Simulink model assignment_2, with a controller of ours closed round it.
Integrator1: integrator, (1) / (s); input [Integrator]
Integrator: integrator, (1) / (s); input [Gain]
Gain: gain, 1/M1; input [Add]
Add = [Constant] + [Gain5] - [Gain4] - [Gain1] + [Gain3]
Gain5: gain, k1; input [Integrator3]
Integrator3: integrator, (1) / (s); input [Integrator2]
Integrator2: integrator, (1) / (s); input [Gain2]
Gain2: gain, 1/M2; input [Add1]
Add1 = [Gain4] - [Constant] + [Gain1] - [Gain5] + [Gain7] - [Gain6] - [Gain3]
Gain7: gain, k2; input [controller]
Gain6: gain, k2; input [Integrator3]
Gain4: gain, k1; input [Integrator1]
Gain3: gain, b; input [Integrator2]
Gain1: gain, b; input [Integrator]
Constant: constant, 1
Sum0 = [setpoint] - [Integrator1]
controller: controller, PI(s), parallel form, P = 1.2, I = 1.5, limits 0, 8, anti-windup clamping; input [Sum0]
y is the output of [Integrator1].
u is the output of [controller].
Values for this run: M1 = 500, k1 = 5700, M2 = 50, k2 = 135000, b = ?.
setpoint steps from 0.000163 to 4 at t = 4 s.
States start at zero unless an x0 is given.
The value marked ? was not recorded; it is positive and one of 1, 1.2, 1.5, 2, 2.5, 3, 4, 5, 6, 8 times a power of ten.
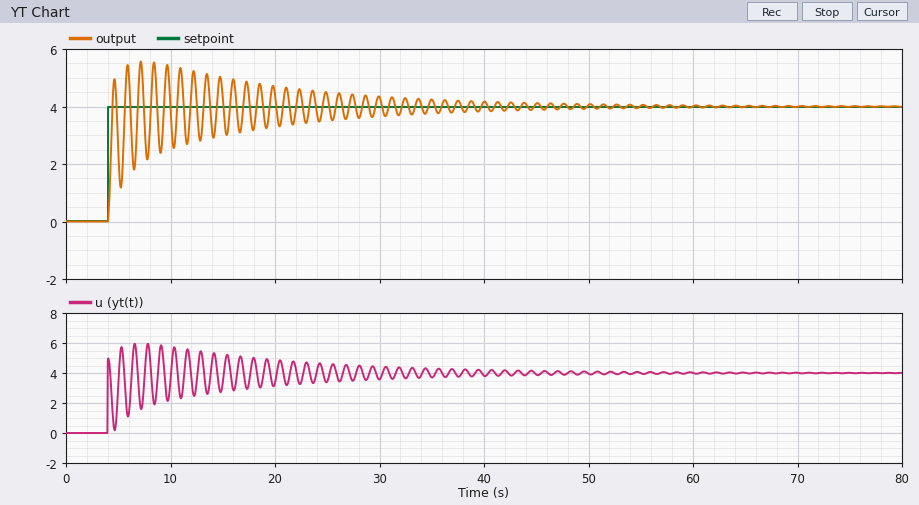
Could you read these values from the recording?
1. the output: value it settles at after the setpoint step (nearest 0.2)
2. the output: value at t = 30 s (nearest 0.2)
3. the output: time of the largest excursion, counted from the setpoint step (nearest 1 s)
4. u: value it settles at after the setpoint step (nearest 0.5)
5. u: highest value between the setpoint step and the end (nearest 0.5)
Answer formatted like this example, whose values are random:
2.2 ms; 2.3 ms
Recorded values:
4.0; 4.4; 3 s; 4.0; 6.0
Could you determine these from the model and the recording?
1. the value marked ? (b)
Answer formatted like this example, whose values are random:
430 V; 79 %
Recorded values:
200
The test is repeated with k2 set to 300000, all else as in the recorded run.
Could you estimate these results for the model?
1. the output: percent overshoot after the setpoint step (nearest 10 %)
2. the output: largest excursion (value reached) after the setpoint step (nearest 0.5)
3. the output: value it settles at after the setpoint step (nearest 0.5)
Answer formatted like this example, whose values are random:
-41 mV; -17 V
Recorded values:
40 %; 5.5; 4.0
